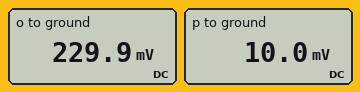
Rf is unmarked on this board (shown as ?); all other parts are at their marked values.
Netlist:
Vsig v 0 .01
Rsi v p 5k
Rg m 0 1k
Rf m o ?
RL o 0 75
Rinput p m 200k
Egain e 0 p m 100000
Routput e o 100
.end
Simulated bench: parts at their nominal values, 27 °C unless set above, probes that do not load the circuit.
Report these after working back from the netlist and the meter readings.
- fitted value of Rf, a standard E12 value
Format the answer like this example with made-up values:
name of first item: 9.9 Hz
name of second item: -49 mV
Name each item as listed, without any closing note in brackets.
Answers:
fitted value of Rf, a standard E12 value: 22 kΩ
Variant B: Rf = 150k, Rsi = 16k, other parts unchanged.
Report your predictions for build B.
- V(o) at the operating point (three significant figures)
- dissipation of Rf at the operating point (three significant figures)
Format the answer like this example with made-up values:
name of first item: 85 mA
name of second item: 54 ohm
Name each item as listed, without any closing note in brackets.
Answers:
V(o) at the operating point: 1.50 V
dissipation of Rf at the operating point: 14.9 µW
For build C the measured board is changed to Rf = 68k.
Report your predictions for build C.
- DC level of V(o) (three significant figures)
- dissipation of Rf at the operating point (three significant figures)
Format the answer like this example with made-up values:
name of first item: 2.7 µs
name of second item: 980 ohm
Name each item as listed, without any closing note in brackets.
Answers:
DC level of V(o): 689 mV
dissipation of Rf at the operating point: 6.78 µW
